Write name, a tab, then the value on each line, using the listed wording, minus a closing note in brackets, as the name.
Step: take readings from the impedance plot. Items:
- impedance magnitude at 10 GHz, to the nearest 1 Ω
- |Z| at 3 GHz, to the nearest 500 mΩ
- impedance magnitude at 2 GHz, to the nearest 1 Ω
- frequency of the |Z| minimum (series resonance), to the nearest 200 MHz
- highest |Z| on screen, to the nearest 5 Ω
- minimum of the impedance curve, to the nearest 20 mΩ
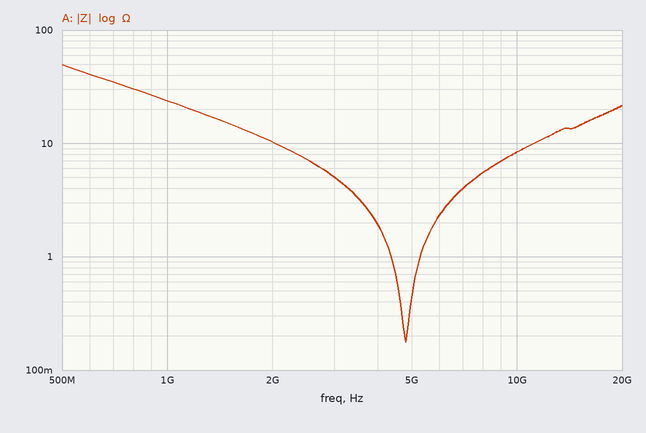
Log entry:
impedance magnitude at 10 GHz, to the nearest 1 Ω	8 Ω
|Z| at 3 GHz, to the nearest 500 mΩ	5.0 Ω
impedance magnitude at 2 GHz, to the nearest 1 Ω	10 Ω
frequency of the |Z| minimum (series resonance), to the nearest 200 MHz	4.8 GHz
highest |Z| on screen, to the nearest 5 Ω	50 Ω
minimum of the impedance curve, to the nearest 20 mΩ	180 mΩ
